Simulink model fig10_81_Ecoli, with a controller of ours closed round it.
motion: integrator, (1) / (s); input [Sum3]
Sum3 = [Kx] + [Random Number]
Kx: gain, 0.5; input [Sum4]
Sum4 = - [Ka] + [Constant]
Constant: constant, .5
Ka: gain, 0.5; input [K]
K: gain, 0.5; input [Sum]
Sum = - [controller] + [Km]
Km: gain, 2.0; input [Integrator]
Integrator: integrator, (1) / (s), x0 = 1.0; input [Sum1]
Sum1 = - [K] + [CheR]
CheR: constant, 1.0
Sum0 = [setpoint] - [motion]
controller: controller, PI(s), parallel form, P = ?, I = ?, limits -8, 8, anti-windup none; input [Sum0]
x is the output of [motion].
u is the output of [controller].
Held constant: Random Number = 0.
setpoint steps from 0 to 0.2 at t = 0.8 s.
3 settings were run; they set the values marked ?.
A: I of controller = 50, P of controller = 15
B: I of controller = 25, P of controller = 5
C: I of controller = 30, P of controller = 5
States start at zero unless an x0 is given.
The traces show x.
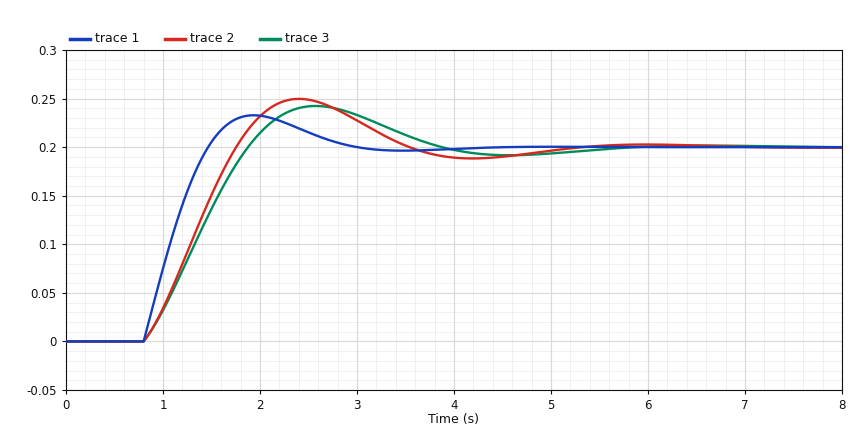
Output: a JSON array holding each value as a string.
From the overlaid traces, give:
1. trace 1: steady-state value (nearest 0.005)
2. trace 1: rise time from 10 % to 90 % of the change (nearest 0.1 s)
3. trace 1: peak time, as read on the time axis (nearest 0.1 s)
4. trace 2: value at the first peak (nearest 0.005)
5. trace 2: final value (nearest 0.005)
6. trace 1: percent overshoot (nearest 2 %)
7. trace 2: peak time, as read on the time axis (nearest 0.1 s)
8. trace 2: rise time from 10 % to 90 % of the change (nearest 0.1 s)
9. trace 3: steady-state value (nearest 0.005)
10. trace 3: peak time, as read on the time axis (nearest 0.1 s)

["0.200", "0.5 s", "1.9 s", "0.250", "0.200", "16 %", "2.4 s", "0.7 s", "0.200", "2.6 s"]
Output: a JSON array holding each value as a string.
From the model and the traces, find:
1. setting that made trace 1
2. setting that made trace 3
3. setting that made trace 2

["A", "B", "C"]
